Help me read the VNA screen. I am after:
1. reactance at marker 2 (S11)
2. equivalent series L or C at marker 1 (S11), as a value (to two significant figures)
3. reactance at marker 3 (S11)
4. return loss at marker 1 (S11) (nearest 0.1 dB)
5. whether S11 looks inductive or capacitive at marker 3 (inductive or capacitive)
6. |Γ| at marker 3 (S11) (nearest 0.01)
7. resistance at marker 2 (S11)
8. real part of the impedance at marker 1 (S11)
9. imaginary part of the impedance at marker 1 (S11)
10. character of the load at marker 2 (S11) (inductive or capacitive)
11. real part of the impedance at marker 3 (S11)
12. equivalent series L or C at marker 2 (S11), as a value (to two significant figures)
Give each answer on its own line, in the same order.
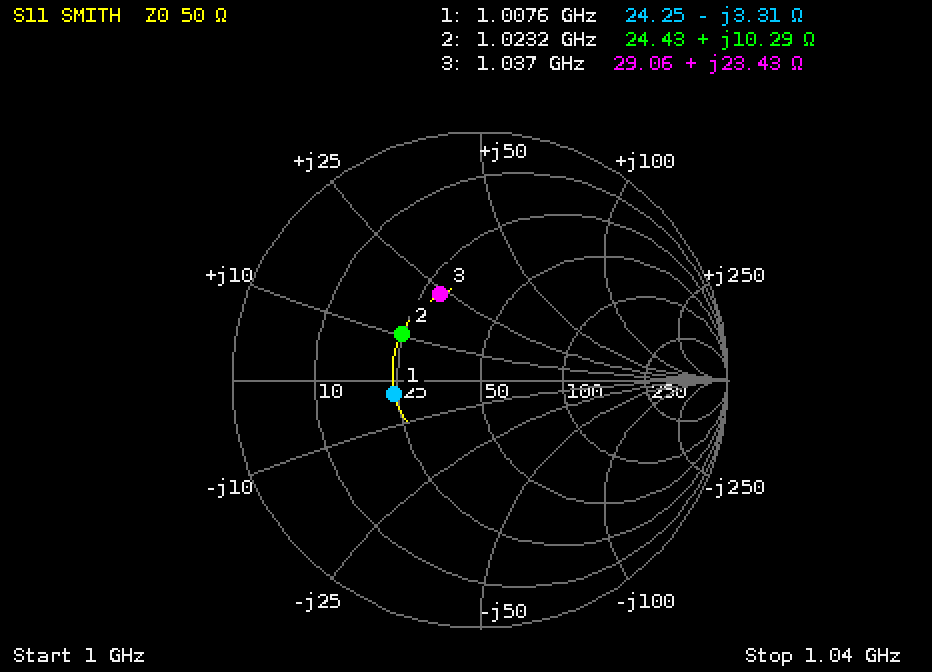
+10.29 Ω
48 pF
+23.43 Ω
9.1 dB
inductive
0.38
24.43 Ω
24.25 Ω
-3.31 Ω
inductive
29.06 Ω
1.6 nH
